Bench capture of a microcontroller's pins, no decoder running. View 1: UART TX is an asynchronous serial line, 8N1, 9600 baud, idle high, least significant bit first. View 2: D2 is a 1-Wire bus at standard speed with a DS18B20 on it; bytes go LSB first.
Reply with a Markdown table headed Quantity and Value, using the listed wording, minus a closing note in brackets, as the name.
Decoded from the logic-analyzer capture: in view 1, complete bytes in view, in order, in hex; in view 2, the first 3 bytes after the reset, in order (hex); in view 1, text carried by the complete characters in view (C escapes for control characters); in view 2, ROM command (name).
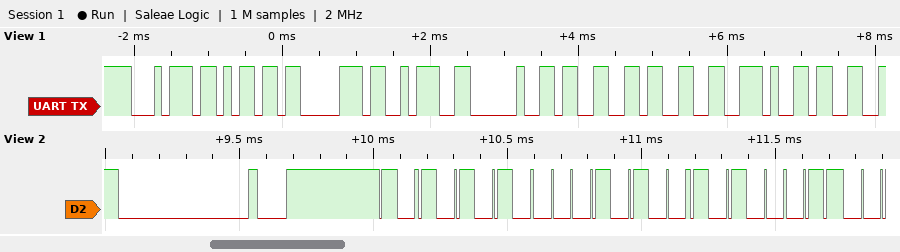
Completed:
| Quantity | Value |
|---|---|
| in view 1, complete bytes in view, in order, in hex | 74 6D 70 3A 20 33 33 2E 33 |
| in view 2, the first 3 bytes after the reset, in order | 55 28 C5 |
| in view 1, text carried by the complete characters in view | "tmp: 33.3" |
| in view 2, ROM command | Match ROM |
